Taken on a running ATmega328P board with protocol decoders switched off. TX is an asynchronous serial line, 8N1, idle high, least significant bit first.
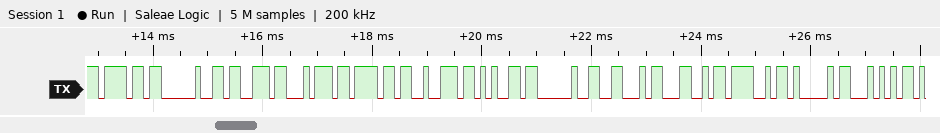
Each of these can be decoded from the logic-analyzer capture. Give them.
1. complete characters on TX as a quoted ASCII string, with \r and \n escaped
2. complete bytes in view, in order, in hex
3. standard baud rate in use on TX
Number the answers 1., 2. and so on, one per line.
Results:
1. "o store FLOAT"
2. 0x6F 0x20 0x73 0x74 0x6F 0x72 0x65 0x20 0x46 0x4C 0x4F 0x41 0x54
3. 9600 baud
